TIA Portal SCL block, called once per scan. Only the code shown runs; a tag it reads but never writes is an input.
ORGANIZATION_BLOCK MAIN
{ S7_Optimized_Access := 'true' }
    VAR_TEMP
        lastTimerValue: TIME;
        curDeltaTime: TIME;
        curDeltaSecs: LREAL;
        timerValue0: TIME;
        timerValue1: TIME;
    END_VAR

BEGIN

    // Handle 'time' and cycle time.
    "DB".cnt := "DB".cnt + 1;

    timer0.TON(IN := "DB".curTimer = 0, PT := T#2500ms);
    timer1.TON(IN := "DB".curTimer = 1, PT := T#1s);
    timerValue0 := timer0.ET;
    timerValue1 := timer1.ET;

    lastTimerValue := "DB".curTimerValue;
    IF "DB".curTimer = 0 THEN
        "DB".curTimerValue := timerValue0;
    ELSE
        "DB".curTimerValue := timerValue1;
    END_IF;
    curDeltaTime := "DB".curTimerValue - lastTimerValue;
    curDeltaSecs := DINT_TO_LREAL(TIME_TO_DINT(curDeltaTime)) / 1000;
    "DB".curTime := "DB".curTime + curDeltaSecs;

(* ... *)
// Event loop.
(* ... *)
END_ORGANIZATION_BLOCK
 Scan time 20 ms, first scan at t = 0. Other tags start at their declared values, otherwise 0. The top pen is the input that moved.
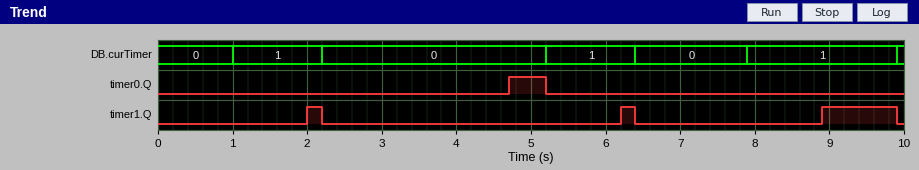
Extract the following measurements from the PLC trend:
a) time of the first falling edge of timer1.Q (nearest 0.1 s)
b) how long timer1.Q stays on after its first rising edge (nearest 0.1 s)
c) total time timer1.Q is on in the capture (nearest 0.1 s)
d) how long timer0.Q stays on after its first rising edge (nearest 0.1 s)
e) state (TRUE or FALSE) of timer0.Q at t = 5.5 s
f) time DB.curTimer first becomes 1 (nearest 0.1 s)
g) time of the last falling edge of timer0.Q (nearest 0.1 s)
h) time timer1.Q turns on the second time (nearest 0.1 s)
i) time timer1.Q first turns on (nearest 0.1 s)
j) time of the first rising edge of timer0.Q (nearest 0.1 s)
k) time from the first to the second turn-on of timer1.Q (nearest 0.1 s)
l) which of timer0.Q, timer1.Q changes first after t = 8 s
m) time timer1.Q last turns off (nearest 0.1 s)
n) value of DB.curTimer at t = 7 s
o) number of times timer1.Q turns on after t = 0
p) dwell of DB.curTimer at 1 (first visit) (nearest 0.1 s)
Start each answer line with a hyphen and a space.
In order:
- 2.2 s
- 0.2 s
- 1.4 s
- 0.5 s
- FALSE
- 1.0 s
- 5.2 s
- 6.2 s
- 2.0 s
- 4.7 s
- 4.2 s
- timer1.Q
- 9.9 s
- 0
- 3
- 1.2 s
